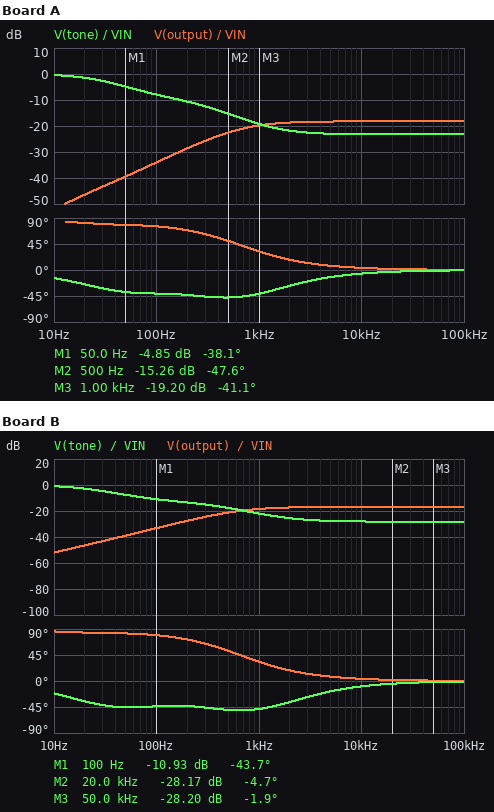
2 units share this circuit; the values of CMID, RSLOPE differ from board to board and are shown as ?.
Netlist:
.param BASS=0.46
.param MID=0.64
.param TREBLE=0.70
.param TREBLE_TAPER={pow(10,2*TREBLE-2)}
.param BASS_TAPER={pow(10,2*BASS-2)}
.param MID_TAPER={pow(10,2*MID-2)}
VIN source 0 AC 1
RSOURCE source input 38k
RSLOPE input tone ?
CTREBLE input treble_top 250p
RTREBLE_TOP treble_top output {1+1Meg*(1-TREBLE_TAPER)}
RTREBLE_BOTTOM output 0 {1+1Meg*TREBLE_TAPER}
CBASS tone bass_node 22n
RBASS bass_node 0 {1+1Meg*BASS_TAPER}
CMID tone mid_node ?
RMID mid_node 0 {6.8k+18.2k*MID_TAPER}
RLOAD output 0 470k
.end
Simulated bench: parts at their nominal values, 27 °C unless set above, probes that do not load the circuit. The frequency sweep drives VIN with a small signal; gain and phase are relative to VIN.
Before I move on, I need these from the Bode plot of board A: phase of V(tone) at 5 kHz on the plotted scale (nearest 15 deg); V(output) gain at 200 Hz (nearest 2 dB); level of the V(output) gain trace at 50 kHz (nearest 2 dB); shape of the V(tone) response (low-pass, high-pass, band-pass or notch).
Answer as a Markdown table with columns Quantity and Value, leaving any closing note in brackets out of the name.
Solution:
| Quantity | Value |
|---|---|
| phase of V(tone) at 5 kHz on the plotted scale | -15 deg |
| V(output) gain at 200 Hz | -28 dB |
| level of the V(output) gain trace at 50 kHz | -18 dB |
| shape of the V(tone) response | low-pass |
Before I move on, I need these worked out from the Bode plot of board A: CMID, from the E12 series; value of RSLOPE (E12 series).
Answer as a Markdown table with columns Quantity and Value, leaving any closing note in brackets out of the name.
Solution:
| Quantity | Value |
|---|---|
| CMID, from the E12 series | 12 nF |
| value of RSLOPE | 82 kΩ |
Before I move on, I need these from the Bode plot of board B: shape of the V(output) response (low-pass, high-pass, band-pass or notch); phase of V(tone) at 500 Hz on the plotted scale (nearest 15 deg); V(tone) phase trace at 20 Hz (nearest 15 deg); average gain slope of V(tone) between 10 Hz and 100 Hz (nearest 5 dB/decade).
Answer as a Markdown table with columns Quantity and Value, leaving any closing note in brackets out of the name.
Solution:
| Quantity | Value |
|---|---|
| shape of the V(output) response | high-pass |
| phase of V(tone) at 500 Hz on the plotted scale | -45 deg |
| V(tone) phase trace at 20 Hz | -30 deg |
| average gain slope of V(tone) between 10 Hz and 100 Hz | -10 dB/decade |
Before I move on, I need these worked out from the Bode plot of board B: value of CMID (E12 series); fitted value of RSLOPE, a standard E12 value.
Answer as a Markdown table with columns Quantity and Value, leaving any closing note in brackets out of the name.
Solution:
| Quantity | Value |
|---|---|
| value of CMID | 8.2 nF |
| fitted value of RSLOPE, a standard E12 value | 180 kΩ |
